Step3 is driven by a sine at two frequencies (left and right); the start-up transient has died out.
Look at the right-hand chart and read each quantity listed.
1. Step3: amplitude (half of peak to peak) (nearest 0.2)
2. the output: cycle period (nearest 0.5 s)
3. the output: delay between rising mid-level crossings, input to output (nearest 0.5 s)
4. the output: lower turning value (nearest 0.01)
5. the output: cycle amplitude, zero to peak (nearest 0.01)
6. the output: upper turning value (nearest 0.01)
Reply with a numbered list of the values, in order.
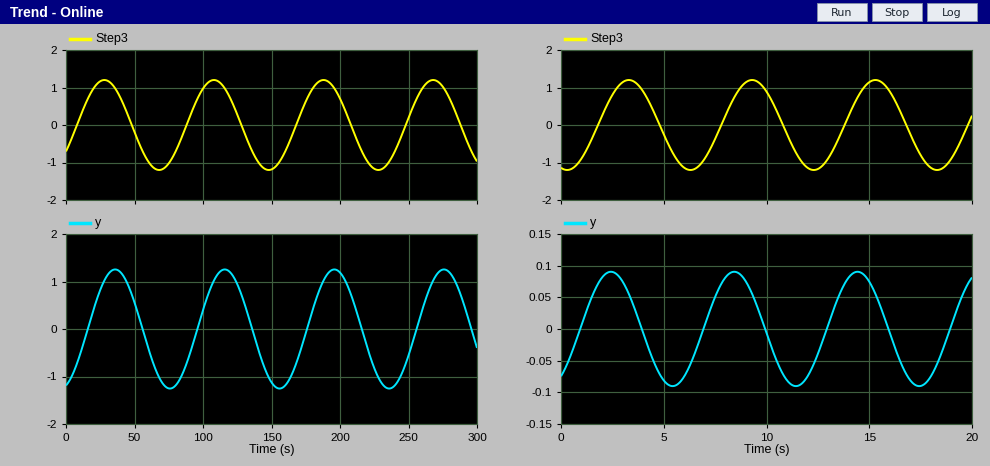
1. 1.2
2. 6.0 s
3. 5.0 s
4. -0.09
5. 0.09
6. 0.09
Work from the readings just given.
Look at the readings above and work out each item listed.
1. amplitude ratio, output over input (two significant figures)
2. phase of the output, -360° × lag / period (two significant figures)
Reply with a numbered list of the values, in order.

1. 0.075
2. -300°
